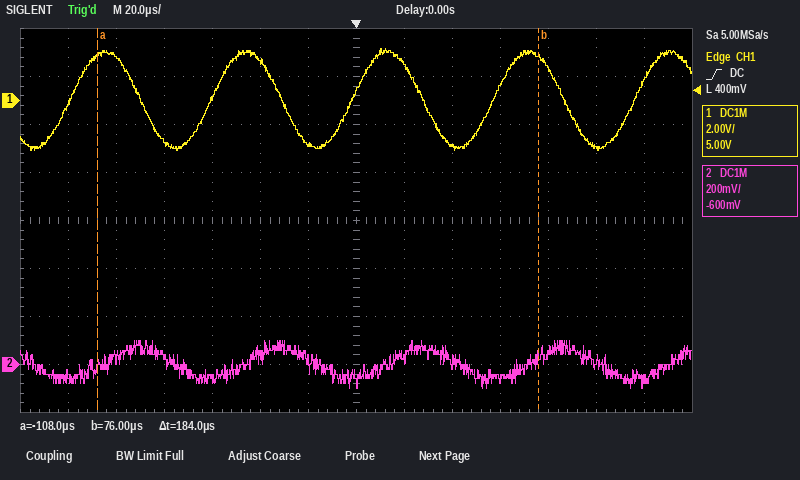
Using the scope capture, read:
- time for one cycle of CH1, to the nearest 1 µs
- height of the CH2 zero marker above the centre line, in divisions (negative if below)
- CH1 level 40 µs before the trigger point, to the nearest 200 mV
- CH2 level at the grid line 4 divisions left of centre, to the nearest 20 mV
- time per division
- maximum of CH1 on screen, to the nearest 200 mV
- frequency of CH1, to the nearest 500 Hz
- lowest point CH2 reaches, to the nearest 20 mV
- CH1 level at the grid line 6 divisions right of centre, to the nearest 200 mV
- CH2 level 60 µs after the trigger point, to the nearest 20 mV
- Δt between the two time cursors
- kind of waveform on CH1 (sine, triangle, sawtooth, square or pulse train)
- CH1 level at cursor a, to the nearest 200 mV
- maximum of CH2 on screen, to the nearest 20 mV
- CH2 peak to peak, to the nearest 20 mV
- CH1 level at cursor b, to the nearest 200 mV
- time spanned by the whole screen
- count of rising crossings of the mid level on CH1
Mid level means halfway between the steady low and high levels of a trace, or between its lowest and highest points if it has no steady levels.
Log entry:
59 µs
-3.0 div
1.6 V
40 mV
20 µs
2.2 V
17.0 kHz
-100 mV
800 mV
-60 mV
184 µs
sine
1.8 V
100 mV
200 mV
1.8 V
280 µs
5
